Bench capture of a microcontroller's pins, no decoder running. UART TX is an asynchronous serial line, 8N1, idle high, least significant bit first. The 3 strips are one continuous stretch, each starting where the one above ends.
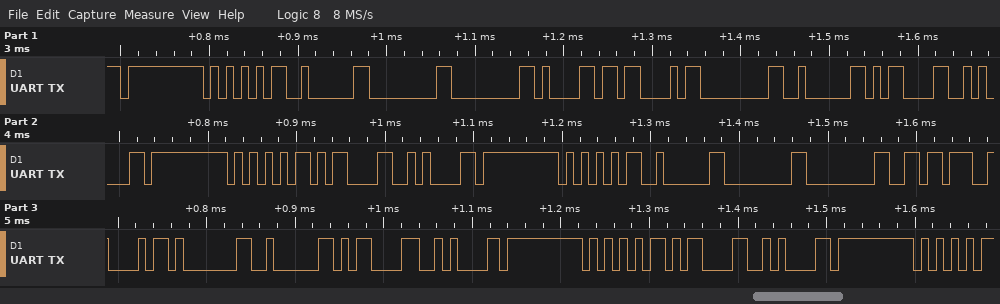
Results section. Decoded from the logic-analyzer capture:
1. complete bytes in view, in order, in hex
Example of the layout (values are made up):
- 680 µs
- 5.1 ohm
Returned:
- FF 55 02 00 00 61 43 00 02 0D 0A FF 55 0D 0A FF 55 02 00 00 B6 42 01 02 0D 0A FF 55 0D 0A FF 55
